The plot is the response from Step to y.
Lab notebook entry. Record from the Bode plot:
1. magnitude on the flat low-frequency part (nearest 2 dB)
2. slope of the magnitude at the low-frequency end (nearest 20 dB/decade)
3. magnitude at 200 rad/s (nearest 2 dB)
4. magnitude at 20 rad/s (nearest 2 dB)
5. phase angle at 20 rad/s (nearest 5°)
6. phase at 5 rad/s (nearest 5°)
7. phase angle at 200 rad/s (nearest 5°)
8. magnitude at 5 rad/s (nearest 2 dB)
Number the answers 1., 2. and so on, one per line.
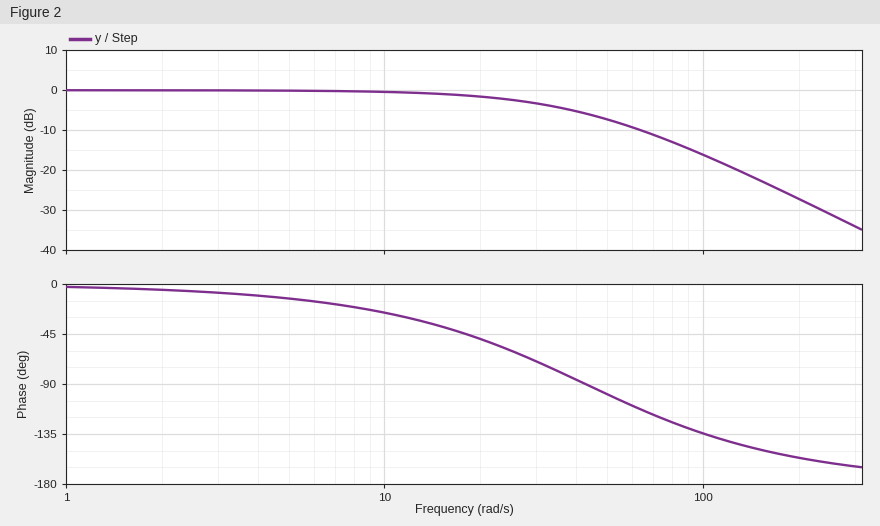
1. 0 dB
2. 0 dB/decade
3. -28 dB
4. -2 dB
5. -50°
6. -15°
7. -155°
8. 0 dB
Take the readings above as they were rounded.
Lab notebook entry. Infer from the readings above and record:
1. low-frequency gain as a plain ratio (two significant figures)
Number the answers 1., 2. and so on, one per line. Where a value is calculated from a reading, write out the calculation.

1. 10^(0 / 20) = 1.0
